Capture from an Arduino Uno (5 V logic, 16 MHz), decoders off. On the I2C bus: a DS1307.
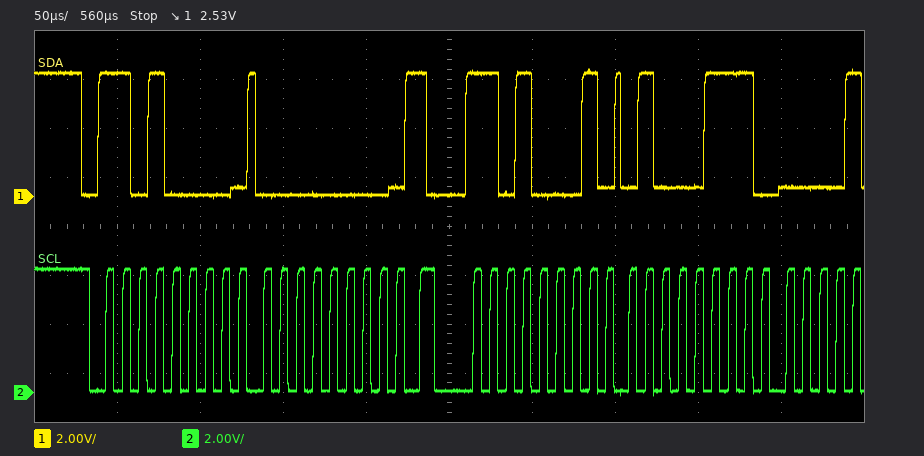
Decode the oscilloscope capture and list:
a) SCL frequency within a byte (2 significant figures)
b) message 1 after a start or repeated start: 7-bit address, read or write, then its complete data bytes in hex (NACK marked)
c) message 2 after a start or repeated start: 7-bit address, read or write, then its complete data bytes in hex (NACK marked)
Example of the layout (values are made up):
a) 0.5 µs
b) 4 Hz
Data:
a) 100 kHz
b) 0x68 write: 00
c) 0x68 read: 47
